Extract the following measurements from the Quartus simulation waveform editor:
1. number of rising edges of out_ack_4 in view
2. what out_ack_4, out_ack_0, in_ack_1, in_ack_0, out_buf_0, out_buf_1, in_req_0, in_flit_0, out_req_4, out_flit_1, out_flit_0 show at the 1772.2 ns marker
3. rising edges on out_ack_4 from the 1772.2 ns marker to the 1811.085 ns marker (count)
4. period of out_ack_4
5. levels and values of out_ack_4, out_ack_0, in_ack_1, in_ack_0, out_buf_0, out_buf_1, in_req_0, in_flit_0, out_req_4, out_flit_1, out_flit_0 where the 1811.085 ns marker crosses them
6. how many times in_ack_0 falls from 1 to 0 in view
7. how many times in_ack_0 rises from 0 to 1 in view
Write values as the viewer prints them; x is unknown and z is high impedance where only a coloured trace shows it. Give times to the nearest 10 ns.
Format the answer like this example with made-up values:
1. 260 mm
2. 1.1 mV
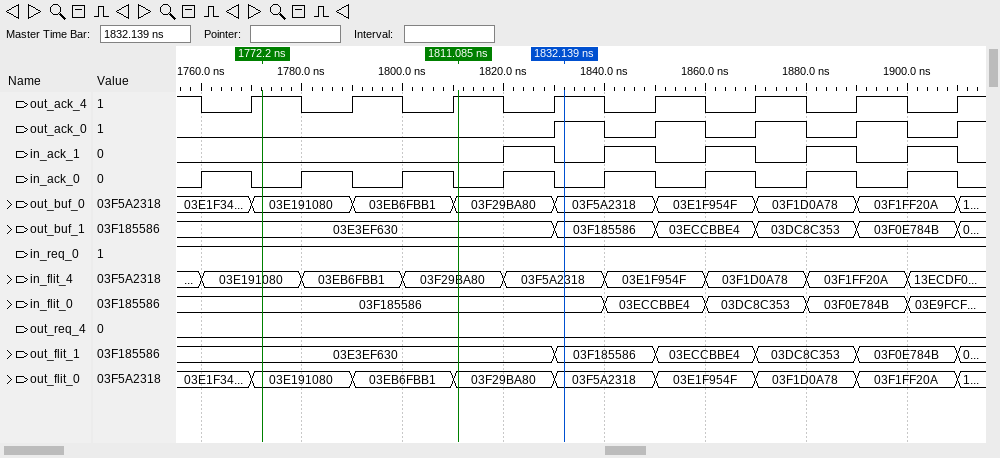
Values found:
1. 8
2. out_ack_4=1, out_ack_0=0, in_ack_1=0, in_ack_0=0, out_buf_0=03E191080, out_buf_1=03E3EF630, in_req_0=1, in_flit_0=03F185586, out_req_4=0, out_flit_1=03E3EF630, out_flit_0=03E191080
3. 2
4. 20 ns
5. out_ack_4=1, out_ack_0=0, in_ack_1=0, in_ack_0=0, out_buf_0=03F29BA80, out_buf_1=03E3EF630, in_req_0=1, in_flit_0=03F185586, out_req_4=0, out_flit_1=03E3EF630, out_flit_0=03F29BA80
6. 8
7. 8
